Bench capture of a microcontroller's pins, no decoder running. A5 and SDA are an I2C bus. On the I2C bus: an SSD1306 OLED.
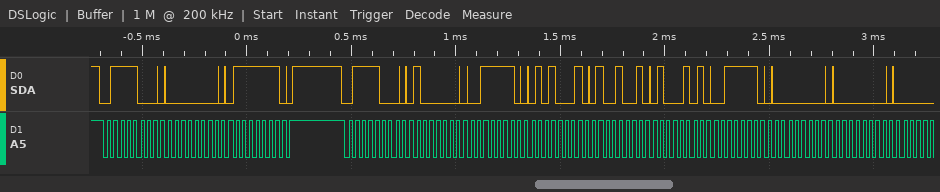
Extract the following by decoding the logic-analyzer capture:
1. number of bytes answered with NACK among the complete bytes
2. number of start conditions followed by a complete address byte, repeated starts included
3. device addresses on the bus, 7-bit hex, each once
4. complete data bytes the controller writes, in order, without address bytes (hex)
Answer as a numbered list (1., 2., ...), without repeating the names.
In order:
1. 0
2. 2
3. 0x3C
4. 00 7F 40 3E 51 49 45 3E 00 00
